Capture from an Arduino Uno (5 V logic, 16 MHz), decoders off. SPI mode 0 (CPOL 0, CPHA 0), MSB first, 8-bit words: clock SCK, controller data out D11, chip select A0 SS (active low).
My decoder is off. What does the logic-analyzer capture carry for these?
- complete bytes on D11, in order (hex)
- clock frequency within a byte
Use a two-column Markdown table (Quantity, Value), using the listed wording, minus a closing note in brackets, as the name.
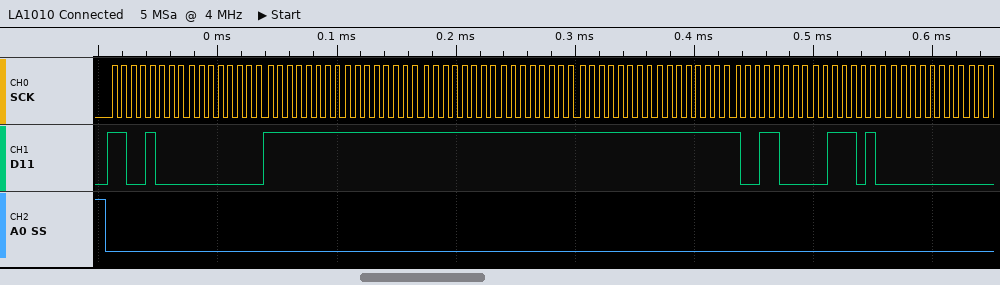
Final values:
| Quantity | Value |
|---|---|
| complete bytes on D11, in order | 0xC8 0x00 0xFF 0xFF 0xFF 0xFF 0xFF 0xFF 0x98 0x3A 0x00 |
| clock frequency within a byte | 125 kHz |
